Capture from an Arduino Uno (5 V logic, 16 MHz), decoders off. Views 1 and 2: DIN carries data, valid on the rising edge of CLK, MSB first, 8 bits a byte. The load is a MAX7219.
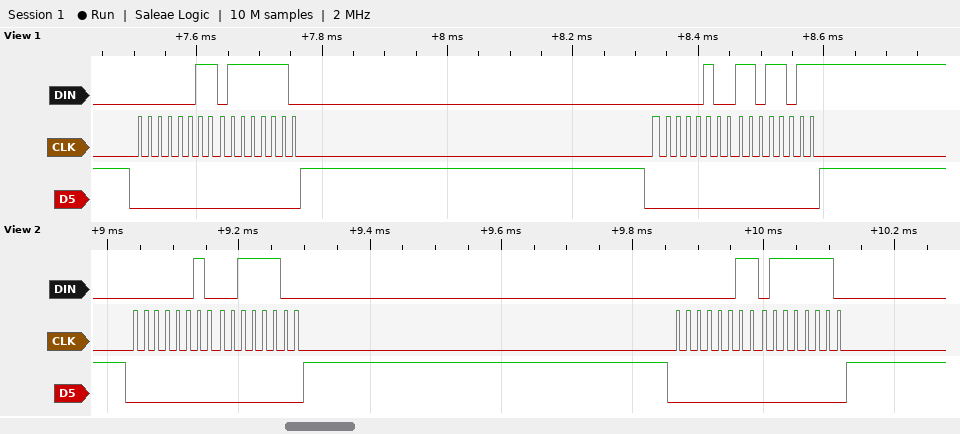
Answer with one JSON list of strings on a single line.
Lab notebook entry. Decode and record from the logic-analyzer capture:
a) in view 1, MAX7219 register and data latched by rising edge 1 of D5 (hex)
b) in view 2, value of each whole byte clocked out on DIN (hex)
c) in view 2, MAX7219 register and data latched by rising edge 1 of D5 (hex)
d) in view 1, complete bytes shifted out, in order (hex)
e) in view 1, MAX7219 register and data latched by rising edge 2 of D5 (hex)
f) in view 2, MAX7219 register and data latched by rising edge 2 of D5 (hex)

["register 0x3, data 0x7E", "02 3C 03 7E", "register 0x2, data 0x3C", "03 7E 04 DB", "register 0x4, data 0xDB", "register 0x3, data 0x7E"]
